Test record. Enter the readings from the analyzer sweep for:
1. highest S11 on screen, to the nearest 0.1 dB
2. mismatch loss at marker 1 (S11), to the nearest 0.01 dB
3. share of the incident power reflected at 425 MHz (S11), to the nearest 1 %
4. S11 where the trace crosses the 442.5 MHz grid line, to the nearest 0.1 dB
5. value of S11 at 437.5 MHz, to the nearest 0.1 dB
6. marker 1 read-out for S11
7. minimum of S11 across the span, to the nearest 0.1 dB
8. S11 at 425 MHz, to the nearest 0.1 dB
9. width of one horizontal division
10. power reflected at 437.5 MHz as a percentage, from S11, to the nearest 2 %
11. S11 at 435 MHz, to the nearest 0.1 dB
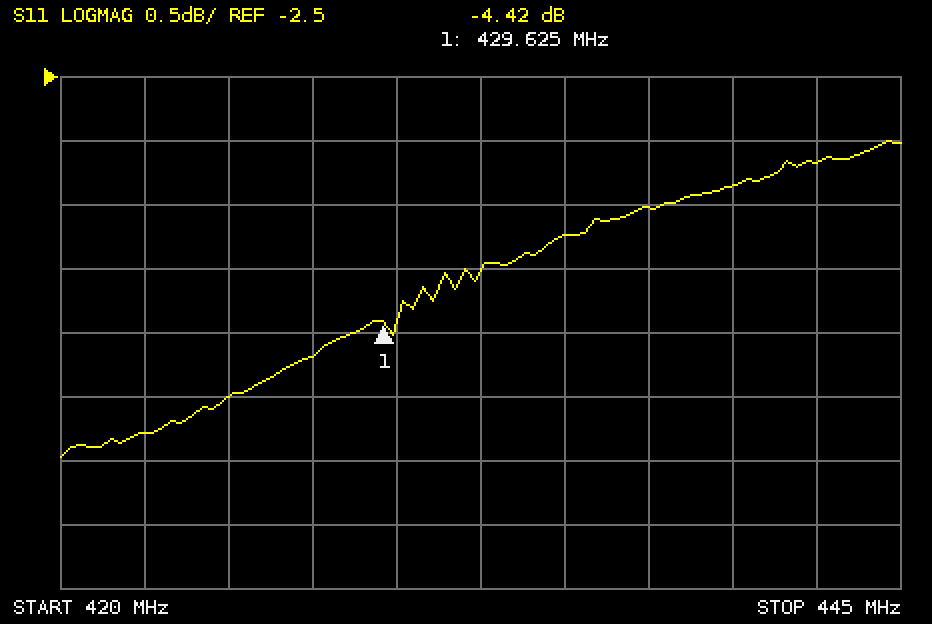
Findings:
-3.0 dB
1.95 dB
32 %
-3.2 dB
-3.5 dB
-4.42 dB
-5.5 dB
-5.0 dB
2.5 MHz
44 %
-3.7 dB
